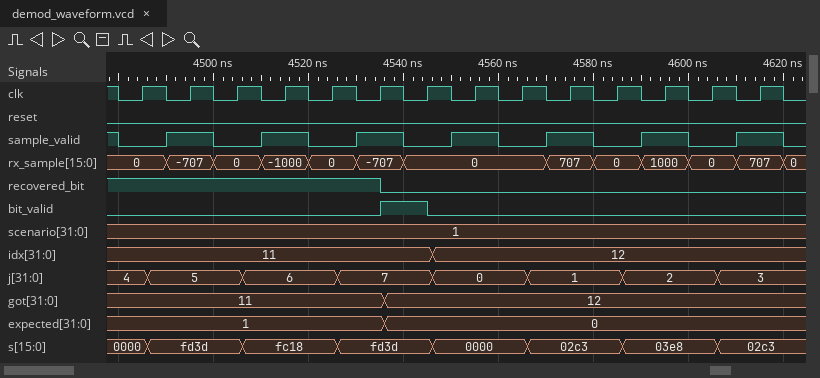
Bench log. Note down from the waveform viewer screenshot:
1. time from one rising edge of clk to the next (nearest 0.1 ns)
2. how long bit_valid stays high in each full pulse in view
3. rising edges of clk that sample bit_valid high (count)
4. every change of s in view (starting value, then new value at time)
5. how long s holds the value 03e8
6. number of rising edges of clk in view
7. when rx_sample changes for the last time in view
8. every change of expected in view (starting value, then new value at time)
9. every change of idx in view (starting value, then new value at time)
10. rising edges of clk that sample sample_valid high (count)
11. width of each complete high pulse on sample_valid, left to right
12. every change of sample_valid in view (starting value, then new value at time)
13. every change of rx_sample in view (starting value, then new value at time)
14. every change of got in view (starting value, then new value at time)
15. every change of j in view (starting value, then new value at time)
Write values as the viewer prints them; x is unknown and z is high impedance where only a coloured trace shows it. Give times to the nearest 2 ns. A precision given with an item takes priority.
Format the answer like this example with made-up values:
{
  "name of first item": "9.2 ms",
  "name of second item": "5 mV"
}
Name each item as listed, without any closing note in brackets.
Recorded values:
{
  "time from one rising edge of clk to the next": "10 ns",
  "how long bit_valid stays high in each full pulse in view": "10 ns",
  "rising edges of clk that sample bit_valid high": "1",
  "every change of s in view": "0000, fd3d at 4486 ns, fc18 at 4506 ns, fd3d at 4526 ns, 0000 at 4546 ns, 02c3 at 4566 ns, 03e8 at 4586 ns, 02c3 at 4606 ns",
  "how long s holds the value 03e8": "20 ns",
  "number of rising edges of clk in view": "14",
  "when rx_sample changes for the last time in view": "4620 ns",
  "every change of expected in view": "1, 0 at 4536 ns",
  "every change of idx in view": "11, 12 at 4546 ns",
  "rising edges of clk that sample sample_valid high": "7",
  "width of each complete high pulse on sample_valid, left to right": "10 ns, 10 ns, 10 ns, 10 ns, 10 ns, 10 ns, 10 ns",
  "every change of sample_valid in view": "1, 0 at 4480 ns, 1 at 4490 ns, 0 at 4500 ns, 1 at 4510 ns, 0 at 4520 ns, 1 at 4530 ns, 0 at 4540 ns, 1 at 4550 ns, 0 at 4560 ns, 1 at 4570 ns, 0 at 4580 ns, 1 at 4590 ns, 0 at 4600 ns, 1 at 4610 ns, 0 at 4620 ns",
  "every change of rx_sample in view": "0, -707 at 4490 ns, 0 at 4500 ns, -1000 at 4510 ns, 0 at 4520 ns, -707 at 4530 ns, 0 at 4540 ns, 707 at 4570 ns, 0 at 4580 ns, 1000 at 4590 ns, 0 at 4600 ns, 707 at 4610 ns, 0 at 4620 ns",
  "every change of got in view": "11, 12 at 4536 ns",
  "every change of j in view": "4, 5 at 4486 ns, 6 at 4506 ns, 7 at 4526 ns, 0 at 4546 ns, 1 at 4566 ns, 2 at 4586 ns, 3 at 4606 ns"
}
